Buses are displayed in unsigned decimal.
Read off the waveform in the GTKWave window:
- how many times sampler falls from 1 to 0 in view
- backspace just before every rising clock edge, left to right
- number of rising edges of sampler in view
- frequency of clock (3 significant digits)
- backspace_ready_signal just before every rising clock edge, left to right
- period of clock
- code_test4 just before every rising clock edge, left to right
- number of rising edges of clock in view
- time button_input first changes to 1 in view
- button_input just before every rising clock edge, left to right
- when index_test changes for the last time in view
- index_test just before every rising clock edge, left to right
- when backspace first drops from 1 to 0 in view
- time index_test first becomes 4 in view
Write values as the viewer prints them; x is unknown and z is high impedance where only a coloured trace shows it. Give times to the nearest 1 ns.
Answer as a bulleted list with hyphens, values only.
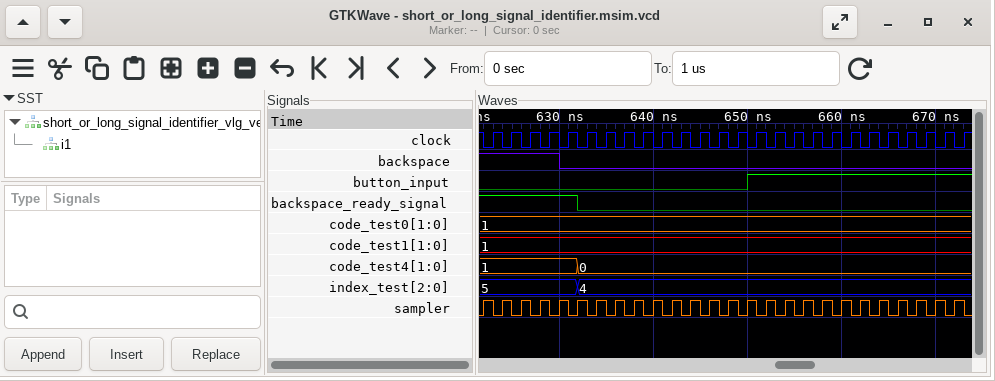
- 26
- 1 1 1 1 0 0 0 0 0 0 0 0 0 0 0 0 0 0 0 0 0 0 0 0 0 0
- 26
- 500 MHz
- 1 1 1 1 1 0 0 0 0 0 0 0 0 0 0 0 0 0 0 0 0 0 0 0 0 0
- 2 ns
- 1, 1, 1, 1, 1, 0, 0, 0, 0, 0, 0, 0, 0, 0, 0, 0, 0, 0, 0, 0, 0, 0, 0, 0, 0, 0
- 26
- 650 ns
- 0 0 0 0 0 0 0 0 0 0 0 0 0 0 1 1 1 1 1 1 1 1 1 1 1 1
- 632 ns
- 5, 5, 5, 5, 5, 4, 4, 4, 4, 4, 4, 4, 4, 4, 4, 4, 4, 4, 4, 4, 4, 4, 4, 4, 4, 4
- 630 ns
- 632 ns
